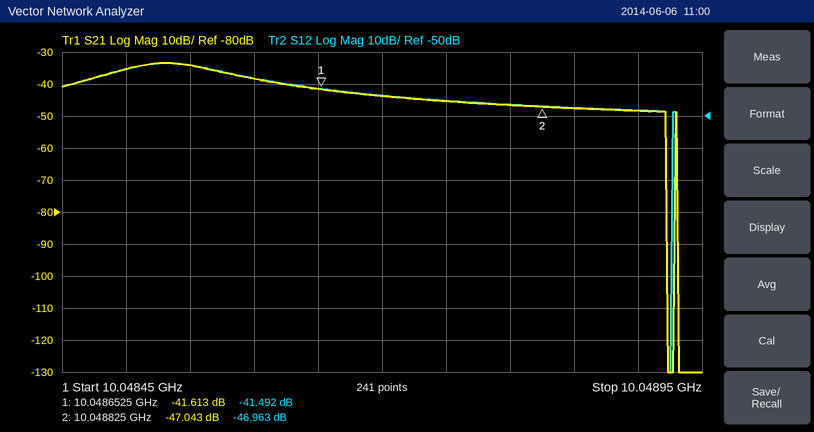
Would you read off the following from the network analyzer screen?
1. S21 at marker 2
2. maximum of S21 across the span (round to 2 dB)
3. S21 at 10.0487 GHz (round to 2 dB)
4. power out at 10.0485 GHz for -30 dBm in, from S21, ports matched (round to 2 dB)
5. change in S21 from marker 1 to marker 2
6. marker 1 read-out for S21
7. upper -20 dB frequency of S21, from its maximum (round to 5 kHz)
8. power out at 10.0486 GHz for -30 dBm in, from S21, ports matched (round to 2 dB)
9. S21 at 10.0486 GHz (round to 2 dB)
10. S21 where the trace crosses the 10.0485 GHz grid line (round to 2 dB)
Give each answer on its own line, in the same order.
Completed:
-47.043 dB
-34 dB
-44 dB
-66 dBm
-5.430 dB
-41.613 dB
10.048920 GHz
-68 dBm
-38 dB
-36 dB
